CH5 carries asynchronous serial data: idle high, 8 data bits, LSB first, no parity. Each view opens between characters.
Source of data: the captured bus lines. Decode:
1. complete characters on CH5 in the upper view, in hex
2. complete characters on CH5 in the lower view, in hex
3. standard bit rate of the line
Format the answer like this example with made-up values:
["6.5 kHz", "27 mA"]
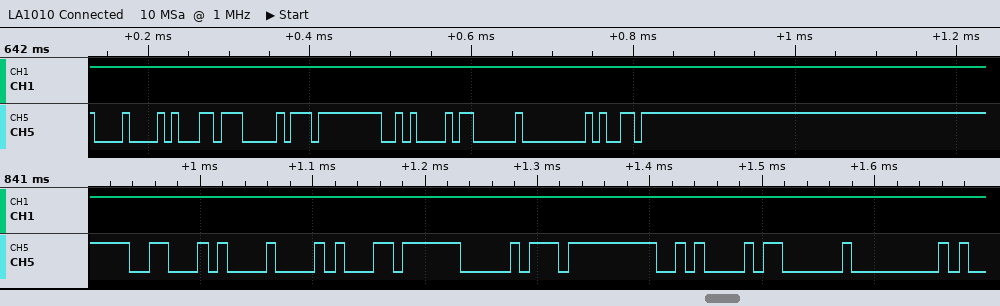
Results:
["08, B1, D0, FF, 0A, 03, 00, D9", "46, 08, B1, D0, FF, 0A, 03, 00", "115200 baud"]
